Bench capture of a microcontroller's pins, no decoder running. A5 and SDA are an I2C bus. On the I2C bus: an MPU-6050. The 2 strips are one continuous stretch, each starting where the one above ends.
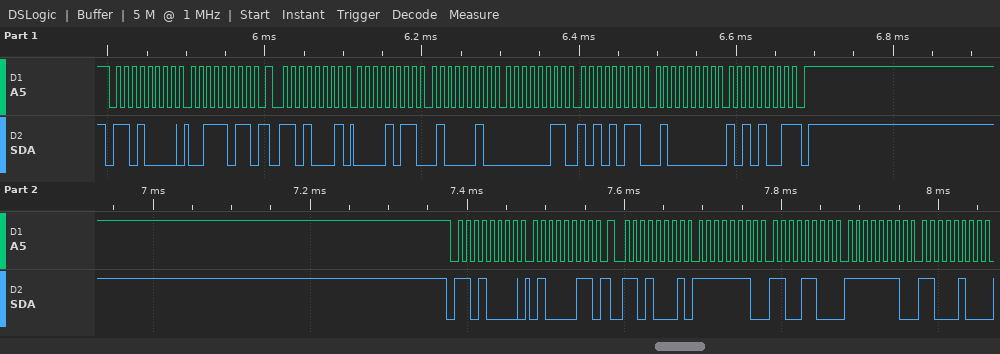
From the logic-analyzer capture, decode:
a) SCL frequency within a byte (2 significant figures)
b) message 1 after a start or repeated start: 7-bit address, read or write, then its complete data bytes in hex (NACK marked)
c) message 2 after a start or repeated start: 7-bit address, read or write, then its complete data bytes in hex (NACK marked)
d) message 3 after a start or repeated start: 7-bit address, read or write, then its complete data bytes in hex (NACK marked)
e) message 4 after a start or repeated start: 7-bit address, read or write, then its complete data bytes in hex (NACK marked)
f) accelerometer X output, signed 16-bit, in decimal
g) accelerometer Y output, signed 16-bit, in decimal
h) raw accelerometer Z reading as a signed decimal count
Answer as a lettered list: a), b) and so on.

a) 100 kHz
b) 0x68 write: 3B
c) 0x68 read: 0B 42 03 AB 40 A9 NACK
d) 0x68 write: 43
e) 0x68 read: FE CC FE C4
f) 2882
g) 939
h) 16553
